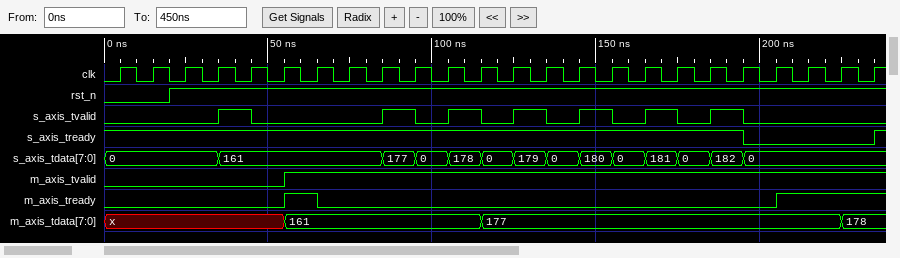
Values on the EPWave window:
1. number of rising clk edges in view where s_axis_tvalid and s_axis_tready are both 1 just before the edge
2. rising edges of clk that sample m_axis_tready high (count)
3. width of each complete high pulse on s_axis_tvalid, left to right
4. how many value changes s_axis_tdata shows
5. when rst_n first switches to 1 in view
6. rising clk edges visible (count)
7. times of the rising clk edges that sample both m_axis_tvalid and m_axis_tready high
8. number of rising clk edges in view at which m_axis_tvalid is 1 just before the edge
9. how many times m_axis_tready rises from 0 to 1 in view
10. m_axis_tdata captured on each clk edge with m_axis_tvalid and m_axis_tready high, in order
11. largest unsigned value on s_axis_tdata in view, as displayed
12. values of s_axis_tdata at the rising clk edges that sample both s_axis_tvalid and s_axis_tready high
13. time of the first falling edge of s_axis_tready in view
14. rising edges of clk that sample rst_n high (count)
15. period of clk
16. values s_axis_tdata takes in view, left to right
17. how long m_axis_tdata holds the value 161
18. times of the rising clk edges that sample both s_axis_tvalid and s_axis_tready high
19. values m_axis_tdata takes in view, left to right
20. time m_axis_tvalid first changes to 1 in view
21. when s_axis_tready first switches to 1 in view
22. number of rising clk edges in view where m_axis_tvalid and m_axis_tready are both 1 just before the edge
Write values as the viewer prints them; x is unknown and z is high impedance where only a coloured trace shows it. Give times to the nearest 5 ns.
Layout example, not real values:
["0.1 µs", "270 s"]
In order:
["7", "4", "10 ns, 10 ns, 10 ns, 10 ns, 10 ns, 10 ns, 10 ns", "13", "20 ns", "24", "65 ns, 215 ns, 225 ns, 235 ns", "18", "2", "161, 177, 177, 178", "182", "161, 177, 178, 179, 180, 181, 182", "195 ns", "22", "10 ns", "0, 161, 177, 0, 178, 0, 179, 0, 180, 0, 181, 0, 182, 0", "60 ns", "45 ns, 95 ns, 115 ns, 135 ns, 155 ns, 175 ns, 195 ns", "x, 161, 177, 178", "55 ns", "235 ns", "4"]
